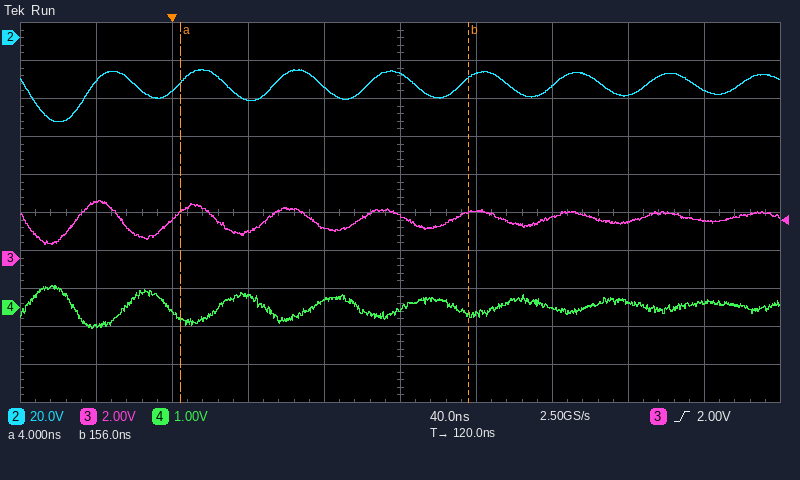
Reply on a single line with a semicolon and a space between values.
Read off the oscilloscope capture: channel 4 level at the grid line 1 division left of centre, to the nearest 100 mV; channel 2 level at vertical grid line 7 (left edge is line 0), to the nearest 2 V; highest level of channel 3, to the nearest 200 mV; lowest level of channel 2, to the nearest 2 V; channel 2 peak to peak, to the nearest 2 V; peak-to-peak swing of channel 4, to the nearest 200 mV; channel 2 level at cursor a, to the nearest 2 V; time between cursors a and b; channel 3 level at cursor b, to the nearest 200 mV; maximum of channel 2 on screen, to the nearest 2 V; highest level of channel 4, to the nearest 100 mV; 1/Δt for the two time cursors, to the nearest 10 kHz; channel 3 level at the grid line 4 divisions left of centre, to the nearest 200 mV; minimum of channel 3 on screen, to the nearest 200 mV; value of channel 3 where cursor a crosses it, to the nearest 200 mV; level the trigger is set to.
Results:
200 mV; -26 V; 3.0 V; -44 V; 28 V; 1.2 V; -24 V; 152 ns; 2.4 V; -16 V; 600 mV; 6.58 MHz; 3.0 V; 800 mV; 2.4 V; 2.00 V
